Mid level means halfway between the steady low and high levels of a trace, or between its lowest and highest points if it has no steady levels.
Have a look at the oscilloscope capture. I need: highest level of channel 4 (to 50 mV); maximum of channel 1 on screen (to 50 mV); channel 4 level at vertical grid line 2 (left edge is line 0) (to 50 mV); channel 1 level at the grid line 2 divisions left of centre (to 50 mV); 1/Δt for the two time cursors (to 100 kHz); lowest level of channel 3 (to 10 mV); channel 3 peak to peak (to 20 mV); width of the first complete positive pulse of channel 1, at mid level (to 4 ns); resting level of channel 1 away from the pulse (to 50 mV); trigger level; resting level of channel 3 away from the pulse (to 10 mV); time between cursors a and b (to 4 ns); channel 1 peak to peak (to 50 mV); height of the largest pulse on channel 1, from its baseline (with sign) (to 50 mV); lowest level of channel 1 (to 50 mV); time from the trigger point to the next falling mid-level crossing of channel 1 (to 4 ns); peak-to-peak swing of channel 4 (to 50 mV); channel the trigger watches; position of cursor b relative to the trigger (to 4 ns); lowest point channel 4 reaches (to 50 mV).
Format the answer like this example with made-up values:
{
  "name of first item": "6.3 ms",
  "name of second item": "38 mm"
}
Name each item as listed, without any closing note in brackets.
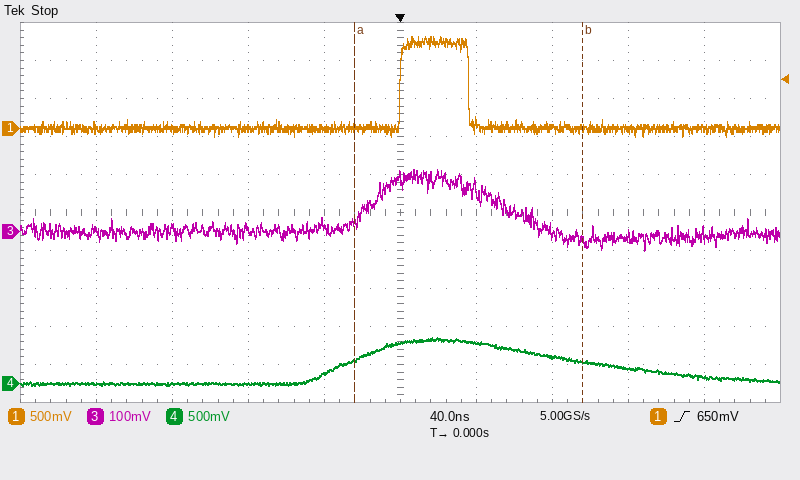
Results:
{
  "highest level of channel 4": "600 mV",
  "maximum of channel 1 on screen": "1.20 V",
  "channel 4 level at vertical grid line 2 (left edge is line 0)": "0 mV",
  "channel 1 level at the grid line 2 divisions left of centre": "0 mV",
  "1/Δt for the two time cursors": "8.3 MHz",
  "lowest level of channel 3": "-50 mV",
  "channel 3 peak to peak": "220 mV",
  "width of the first complete positive pulse of channel 1, at mid level": "36 ns",
  "resting level of channel 1 away from the pulse": "0 mV",
  "trigger level": "650 mV",
  "resting level of channel 3 away from the pulse": "0 mV",
  "time between cursors a and b": "120 ns",
  "channel 1 peak to peak": "1.30 V",
  "height of the largest pulse on channel 1, from its baseline (with sign)": "+1.20 V",
  "lowest level of channel 1": "-100 mV",
  "time from the trigger point to the next falling mid-level crossing of channel 1": "36 ns",
  "peak-to-peak swing of channel 4": "650 mV",
  "channel the trigger watches": "channel 1",
  "position of cursor b relative to the trigger": "+96 ns",
  "lowest point channel 4 reaches": "-50 mV"
}
